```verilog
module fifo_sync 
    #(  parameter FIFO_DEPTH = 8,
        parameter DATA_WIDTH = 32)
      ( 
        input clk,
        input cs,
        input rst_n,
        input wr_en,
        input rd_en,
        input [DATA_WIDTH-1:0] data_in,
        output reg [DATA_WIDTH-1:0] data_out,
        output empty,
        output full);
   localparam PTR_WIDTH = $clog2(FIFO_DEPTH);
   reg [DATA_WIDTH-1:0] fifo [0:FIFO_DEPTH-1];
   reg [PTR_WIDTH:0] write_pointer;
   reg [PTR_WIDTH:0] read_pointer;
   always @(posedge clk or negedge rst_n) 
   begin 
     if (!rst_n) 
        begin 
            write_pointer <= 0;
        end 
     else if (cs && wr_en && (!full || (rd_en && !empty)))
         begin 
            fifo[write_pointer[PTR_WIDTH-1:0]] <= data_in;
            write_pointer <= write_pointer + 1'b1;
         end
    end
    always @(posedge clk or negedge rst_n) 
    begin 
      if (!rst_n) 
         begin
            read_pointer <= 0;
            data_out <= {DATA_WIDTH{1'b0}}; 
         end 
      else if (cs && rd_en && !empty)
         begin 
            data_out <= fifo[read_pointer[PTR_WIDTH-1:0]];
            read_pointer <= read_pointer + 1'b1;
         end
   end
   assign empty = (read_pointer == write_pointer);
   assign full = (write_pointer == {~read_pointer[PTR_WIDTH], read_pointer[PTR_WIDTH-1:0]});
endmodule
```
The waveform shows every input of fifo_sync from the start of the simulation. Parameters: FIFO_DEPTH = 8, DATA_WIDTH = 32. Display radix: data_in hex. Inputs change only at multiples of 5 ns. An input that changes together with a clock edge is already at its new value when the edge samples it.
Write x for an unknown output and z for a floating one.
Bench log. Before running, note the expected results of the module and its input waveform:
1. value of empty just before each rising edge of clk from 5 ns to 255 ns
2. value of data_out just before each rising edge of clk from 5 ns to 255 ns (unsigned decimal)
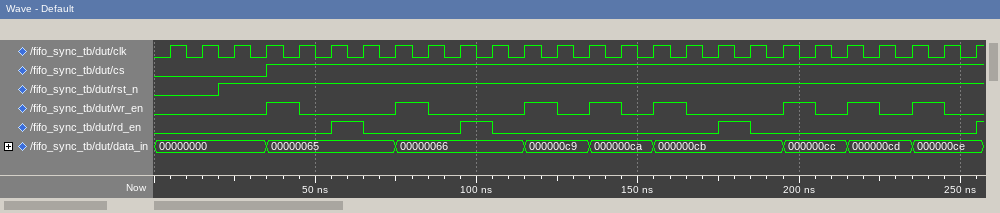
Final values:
1 1 1 1 0 0 1 1 0 0 1 1 0 0 0 0 0 0 0 0 0 0 0 0 0 0
0, 0, 0, 0, 0, 0, 101, 101, 101, 101, 102, 102, 102, 102, 102, 102, 102, 102, 201, 201, 201, 201, 201, 201, 201, 201
